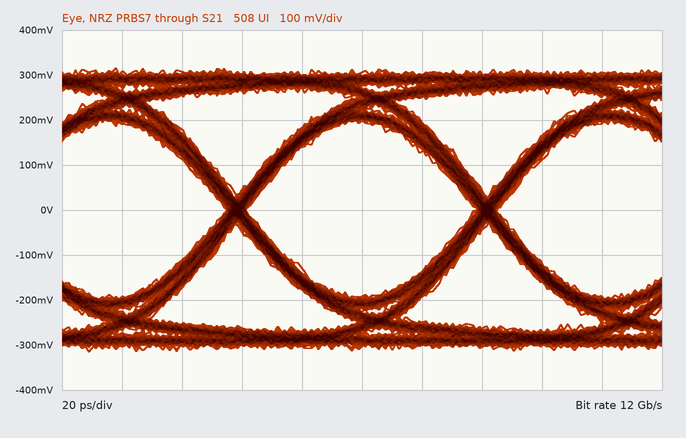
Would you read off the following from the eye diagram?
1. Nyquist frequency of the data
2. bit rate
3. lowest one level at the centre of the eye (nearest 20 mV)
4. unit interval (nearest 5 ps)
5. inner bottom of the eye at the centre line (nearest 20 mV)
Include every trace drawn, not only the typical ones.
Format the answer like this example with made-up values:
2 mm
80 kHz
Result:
6 GHz
12 Gb/s
200 mV
85 ps
-200 mV
